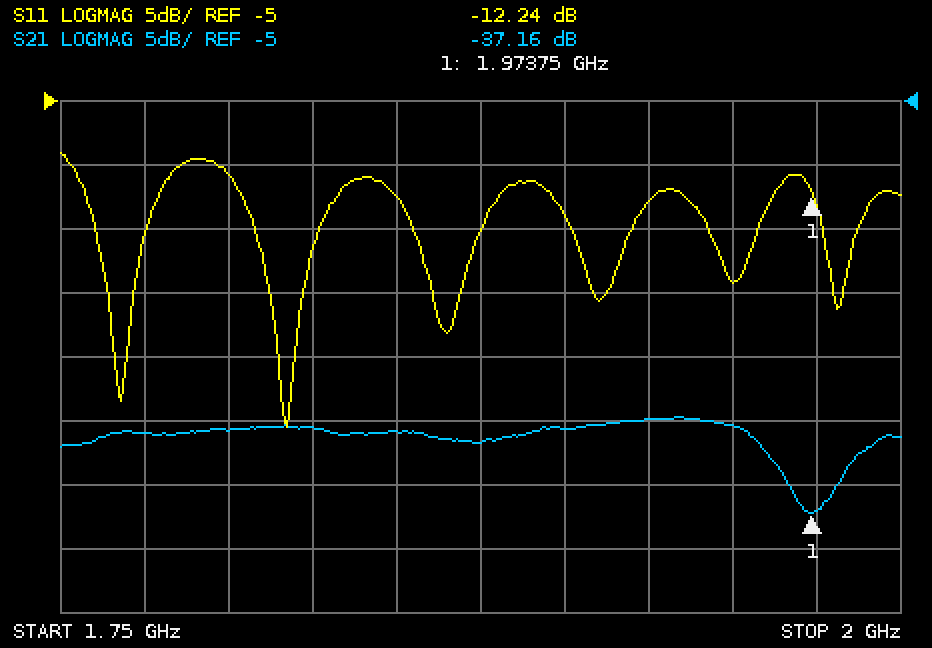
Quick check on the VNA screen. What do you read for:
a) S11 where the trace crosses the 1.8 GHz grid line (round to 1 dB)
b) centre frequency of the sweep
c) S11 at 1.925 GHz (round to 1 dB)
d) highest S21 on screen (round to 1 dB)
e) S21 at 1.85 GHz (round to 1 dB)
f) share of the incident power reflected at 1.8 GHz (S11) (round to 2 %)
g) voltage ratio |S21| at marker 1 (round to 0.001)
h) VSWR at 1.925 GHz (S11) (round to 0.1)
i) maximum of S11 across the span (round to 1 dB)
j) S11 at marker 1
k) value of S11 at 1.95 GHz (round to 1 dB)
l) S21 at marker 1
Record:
-11 dB
1.875 GHz
-13 dB
-30 dB
-31 dB
8 %
0.014
1.6
-9 dB
-12.24 dB
-19 dB
-37.16 dB
